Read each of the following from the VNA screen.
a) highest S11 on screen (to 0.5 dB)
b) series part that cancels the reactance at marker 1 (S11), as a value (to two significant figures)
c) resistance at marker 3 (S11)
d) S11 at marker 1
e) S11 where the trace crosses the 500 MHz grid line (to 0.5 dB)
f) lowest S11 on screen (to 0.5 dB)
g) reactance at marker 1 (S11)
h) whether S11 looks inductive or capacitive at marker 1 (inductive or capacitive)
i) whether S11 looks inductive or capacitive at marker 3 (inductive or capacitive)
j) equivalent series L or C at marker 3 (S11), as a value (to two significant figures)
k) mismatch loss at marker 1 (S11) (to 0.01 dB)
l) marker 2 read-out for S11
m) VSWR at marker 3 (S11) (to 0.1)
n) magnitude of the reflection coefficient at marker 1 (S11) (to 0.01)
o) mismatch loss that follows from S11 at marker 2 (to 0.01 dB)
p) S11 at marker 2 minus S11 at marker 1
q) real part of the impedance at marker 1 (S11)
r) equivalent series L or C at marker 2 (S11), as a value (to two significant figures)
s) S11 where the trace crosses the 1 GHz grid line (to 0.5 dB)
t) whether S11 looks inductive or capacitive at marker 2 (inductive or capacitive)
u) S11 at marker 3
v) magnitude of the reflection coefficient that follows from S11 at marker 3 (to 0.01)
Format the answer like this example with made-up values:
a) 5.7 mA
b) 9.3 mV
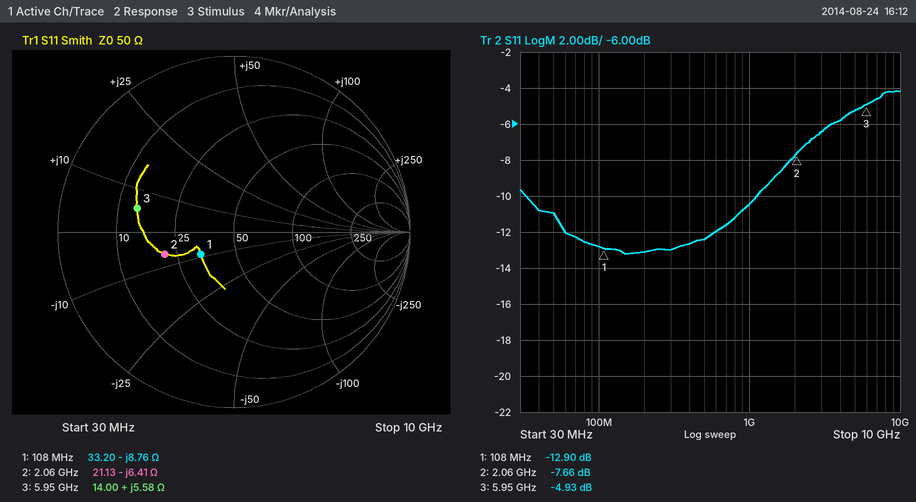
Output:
a) -4.0 dB
b) 13 nH
c) 14.00 Ω
d) -12.90 dB
e) -12.5 dB
f) -13.0 dB
g) -8.76 Ω
h) capacitive
i) inductive
j) 150 pH
k) 0.23 dB
l) -7.66 dB
m) 3.6
n) 0.23
o) 0.82 dB
p) 5.24 dB
q) 33.20 Ω
r) 12 pF
s) -10.5 dB
t) capacitive
u) -4.93 dB
v) 0.57
